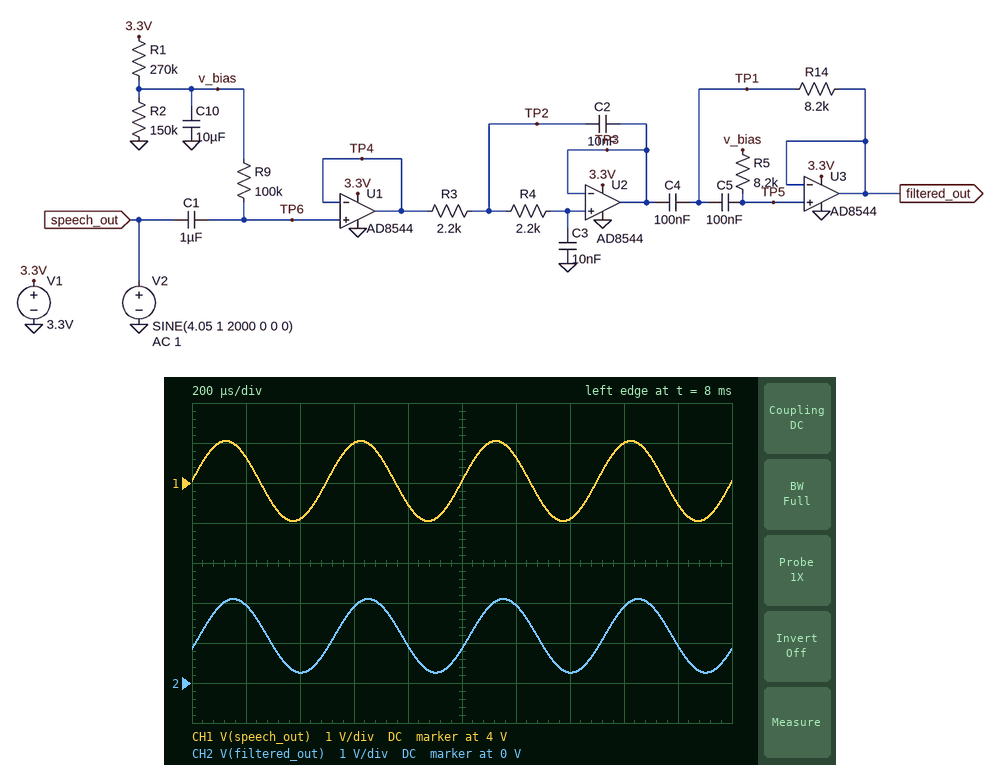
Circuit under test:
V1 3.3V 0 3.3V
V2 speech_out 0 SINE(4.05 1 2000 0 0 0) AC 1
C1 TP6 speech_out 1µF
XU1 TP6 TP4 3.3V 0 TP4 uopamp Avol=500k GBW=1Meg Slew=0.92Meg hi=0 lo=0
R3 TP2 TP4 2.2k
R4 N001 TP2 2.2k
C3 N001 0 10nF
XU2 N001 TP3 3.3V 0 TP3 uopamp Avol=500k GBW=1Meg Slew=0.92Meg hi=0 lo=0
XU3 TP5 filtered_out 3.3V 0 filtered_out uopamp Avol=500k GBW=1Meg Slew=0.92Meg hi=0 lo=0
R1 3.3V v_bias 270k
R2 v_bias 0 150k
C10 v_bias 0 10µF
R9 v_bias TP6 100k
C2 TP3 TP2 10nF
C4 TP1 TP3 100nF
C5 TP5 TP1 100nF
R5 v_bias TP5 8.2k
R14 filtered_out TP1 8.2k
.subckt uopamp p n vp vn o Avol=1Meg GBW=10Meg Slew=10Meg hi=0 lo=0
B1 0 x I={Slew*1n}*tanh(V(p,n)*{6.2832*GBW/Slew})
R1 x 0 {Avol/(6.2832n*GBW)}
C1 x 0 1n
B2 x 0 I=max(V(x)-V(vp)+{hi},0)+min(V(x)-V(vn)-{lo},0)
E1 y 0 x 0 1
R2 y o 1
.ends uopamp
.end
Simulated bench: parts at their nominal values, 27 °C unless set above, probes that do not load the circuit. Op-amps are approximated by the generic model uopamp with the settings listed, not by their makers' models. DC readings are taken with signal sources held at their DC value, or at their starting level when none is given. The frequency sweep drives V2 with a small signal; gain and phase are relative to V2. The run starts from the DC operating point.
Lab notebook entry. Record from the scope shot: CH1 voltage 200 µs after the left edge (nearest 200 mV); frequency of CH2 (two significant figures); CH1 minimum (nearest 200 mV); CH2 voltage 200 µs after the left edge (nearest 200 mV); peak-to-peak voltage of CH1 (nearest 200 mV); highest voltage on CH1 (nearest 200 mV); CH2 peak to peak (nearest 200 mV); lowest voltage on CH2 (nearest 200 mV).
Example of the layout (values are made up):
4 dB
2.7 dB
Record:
4.6 V
2.0 kHz
3.0 V
2.0 V
2.0 V
5.0 V
1.8 V
200 mV
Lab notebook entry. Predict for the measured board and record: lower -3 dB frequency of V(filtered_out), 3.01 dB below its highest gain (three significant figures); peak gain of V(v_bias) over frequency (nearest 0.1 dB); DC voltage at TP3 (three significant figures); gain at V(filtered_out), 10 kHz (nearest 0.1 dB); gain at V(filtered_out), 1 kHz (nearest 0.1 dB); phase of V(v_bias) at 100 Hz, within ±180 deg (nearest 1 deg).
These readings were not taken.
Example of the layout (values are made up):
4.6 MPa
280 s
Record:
280 Hz
-21.6 dB
1.18 V
-9.3 dB
-0.5 dB
12 deg
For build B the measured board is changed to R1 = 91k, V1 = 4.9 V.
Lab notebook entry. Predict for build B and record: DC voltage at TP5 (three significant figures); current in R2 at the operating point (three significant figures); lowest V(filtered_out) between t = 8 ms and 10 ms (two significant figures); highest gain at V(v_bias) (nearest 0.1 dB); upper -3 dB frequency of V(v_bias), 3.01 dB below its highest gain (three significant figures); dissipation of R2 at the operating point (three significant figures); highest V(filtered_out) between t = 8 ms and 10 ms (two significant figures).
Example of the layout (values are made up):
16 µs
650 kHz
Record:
3.05 V
20.3 µA
2.1 V
-22.1 dB
2.23 Hz
62.0 µW
4.0 V
